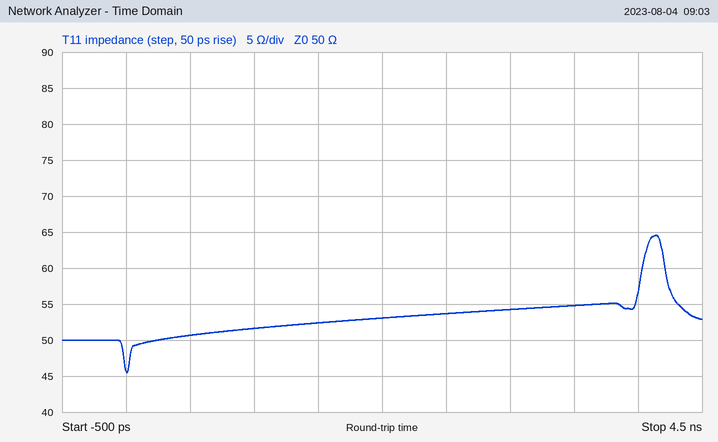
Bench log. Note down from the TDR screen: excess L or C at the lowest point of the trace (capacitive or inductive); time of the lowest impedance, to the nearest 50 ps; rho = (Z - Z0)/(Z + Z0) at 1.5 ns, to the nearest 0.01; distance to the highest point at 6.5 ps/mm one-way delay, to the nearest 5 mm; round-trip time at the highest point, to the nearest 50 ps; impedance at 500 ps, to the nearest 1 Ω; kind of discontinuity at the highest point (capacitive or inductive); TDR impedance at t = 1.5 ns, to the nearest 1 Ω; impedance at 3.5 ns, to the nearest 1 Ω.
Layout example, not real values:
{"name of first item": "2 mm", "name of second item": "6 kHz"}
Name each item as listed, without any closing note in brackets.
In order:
{"excess L or C at the lowest point of the trace": "capacitive", "time of the lowest impedance, to the nearest 50 ps": "0 ps", "rho = (Z - Z0)/(Z + Z0) at 1.5 ns, to the nearest 0.01": "+0.02", "distance to the highest point at 6.5 ps/mm one-way delay, to the nearest 5 mm": "320 mm", "round-trip time at the highest point, to the nearest 50 ps": "4.15 ns", "impedance at 500 ps, to the nearest 1 Ω": "51 Ω", "kind of discontinuity at the highest point": "inductive", "TDR impedance at t = 1.5 ns, to the nearest 1 Ω": "52 Ω", "impedance at 3.5 ns, to the nearest 1 Ω": "55 Ω"}
